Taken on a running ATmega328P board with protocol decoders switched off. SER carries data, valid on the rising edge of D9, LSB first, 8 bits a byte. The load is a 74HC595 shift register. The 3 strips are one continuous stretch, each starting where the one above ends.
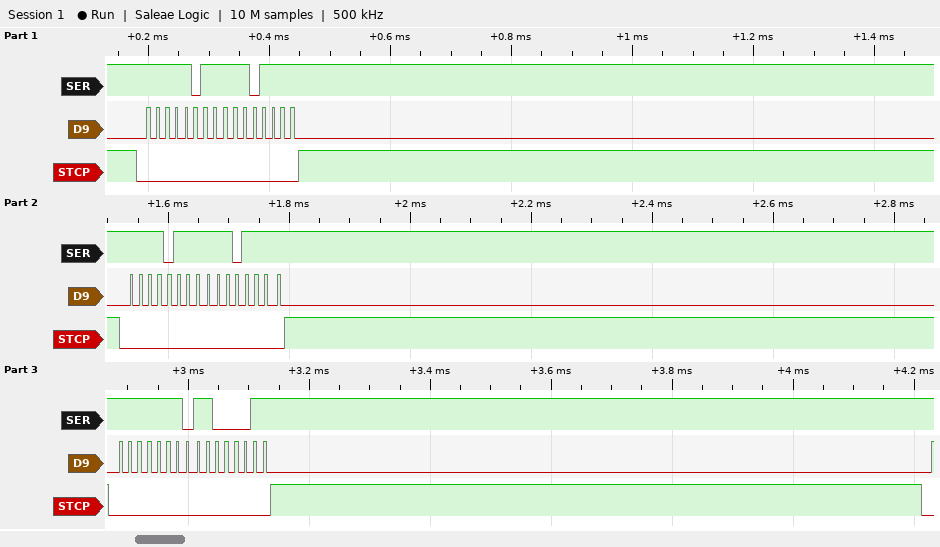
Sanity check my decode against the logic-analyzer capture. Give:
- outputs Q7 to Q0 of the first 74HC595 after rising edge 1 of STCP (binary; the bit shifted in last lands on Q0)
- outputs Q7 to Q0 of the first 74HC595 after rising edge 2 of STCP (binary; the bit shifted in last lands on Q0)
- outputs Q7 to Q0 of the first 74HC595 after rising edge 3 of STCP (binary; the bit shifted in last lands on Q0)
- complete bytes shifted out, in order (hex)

11101111
11101111
11000011
DF F7 EF F7 7F C3
